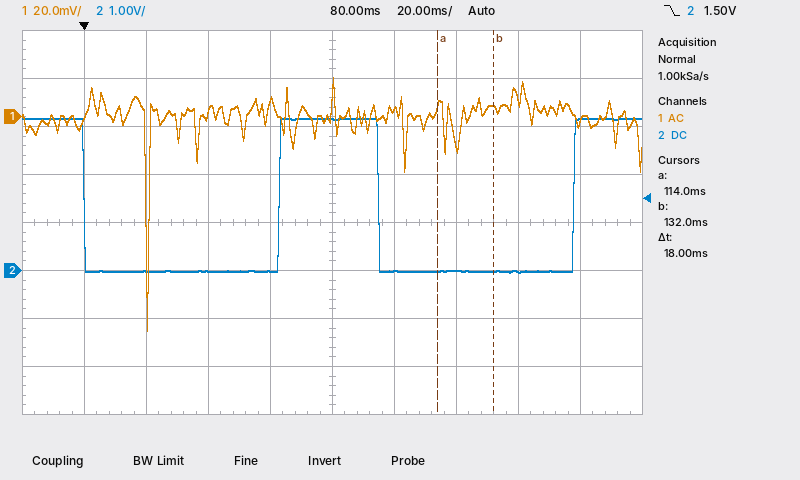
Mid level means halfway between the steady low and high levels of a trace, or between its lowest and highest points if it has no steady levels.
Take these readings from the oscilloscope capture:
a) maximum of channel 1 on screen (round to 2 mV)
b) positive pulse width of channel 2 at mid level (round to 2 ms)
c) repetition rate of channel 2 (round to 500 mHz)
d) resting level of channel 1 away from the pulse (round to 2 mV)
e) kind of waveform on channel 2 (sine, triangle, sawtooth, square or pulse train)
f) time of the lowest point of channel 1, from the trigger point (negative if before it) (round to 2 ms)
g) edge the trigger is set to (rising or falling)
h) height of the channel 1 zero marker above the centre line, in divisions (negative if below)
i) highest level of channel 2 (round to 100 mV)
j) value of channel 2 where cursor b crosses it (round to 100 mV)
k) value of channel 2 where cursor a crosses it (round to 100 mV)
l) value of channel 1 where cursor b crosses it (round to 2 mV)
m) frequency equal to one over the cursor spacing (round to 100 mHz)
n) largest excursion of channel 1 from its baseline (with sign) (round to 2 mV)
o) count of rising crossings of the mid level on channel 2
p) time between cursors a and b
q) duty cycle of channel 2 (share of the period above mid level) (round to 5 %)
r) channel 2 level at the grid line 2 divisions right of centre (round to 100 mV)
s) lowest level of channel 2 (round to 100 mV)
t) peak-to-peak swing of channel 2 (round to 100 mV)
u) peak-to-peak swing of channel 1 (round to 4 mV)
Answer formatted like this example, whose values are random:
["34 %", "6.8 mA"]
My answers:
["16 mV", "32 ms", "10.5 Hz", "0 mV", "pulse train", "+20 ms", "falling", "+2.2 div", "3.2 V", "0.0 V", "0.0 V", "4 mV", "55.6 Hz", "-90 mV", "2", "18 ms", "35 %", "0.0 V", "0.0 V", "3.2 V", "104 mV"]
